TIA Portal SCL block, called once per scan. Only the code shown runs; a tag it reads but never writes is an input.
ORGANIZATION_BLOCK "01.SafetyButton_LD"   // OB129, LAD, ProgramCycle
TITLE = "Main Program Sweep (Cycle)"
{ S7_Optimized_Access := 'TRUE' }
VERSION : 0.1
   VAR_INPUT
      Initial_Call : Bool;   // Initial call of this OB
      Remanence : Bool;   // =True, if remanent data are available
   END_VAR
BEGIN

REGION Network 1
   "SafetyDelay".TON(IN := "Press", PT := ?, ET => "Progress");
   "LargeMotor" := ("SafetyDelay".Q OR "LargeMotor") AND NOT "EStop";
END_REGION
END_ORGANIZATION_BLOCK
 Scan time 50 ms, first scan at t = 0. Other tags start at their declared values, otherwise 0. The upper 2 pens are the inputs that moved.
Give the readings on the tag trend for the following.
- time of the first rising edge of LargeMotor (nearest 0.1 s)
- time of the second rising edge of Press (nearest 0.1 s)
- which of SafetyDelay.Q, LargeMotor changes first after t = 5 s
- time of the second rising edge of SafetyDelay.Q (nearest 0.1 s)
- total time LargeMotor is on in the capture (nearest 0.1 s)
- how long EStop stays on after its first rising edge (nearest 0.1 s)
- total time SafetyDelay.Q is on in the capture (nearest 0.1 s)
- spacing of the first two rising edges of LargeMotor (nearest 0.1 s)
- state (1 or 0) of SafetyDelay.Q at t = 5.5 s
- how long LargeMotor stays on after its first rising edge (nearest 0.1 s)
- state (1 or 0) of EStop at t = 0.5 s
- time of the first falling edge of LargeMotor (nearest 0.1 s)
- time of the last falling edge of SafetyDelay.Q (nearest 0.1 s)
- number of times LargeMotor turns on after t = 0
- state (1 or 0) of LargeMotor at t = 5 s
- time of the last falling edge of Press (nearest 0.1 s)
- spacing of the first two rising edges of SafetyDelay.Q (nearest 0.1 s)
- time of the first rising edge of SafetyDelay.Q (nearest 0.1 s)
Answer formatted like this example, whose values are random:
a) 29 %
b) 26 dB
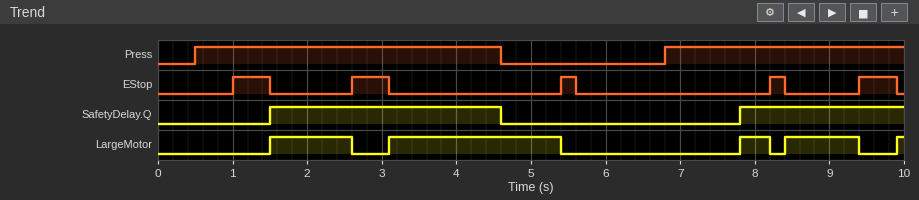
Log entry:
a) 1.5 s
b) 6.8 s
c) LargeMotor
d) 7.8 s
e) 4.9 s
f) 0.5 s
g) 5.3 s
h) 1.6 s
i) 0
j) 1.1 s
k) 0
l) 2.6 s
m) 4.6 s
n) 5
o) 1
p) 4.6 s
q) 6.3 s
r) 1.5 s
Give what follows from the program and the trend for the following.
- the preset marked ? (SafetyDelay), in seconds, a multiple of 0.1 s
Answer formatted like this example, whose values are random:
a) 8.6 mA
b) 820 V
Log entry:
a) 1.0 s
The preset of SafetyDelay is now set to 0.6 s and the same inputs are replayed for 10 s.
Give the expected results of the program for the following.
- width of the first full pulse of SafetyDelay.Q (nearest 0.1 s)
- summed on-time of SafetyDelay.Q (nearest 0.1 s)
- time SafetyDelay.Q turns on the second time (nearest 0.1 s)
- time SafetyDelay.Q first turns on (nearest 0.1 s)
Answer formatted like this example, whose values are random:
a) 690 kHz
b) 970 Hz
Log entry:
a) 3.5 s
b) 6.1 s
c) 7.4 s
d) 1.1 s
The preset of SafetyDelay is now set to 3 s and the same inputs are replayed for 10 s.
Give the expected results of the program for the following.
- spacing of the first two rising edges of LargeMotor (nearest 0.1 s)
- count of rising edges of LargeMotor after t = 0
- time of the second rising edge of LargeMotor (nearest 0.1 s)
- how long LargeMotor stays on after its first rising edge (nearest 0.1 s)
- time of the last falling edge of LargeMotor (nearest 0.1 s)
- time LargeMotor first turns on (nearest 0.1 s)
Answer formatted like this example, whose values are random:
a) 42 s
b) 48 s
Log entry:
a) 6.4 s
b) 2
c) 9.9 s
d) 1.9 s
e) 5.4 s
f) 3.5 s
